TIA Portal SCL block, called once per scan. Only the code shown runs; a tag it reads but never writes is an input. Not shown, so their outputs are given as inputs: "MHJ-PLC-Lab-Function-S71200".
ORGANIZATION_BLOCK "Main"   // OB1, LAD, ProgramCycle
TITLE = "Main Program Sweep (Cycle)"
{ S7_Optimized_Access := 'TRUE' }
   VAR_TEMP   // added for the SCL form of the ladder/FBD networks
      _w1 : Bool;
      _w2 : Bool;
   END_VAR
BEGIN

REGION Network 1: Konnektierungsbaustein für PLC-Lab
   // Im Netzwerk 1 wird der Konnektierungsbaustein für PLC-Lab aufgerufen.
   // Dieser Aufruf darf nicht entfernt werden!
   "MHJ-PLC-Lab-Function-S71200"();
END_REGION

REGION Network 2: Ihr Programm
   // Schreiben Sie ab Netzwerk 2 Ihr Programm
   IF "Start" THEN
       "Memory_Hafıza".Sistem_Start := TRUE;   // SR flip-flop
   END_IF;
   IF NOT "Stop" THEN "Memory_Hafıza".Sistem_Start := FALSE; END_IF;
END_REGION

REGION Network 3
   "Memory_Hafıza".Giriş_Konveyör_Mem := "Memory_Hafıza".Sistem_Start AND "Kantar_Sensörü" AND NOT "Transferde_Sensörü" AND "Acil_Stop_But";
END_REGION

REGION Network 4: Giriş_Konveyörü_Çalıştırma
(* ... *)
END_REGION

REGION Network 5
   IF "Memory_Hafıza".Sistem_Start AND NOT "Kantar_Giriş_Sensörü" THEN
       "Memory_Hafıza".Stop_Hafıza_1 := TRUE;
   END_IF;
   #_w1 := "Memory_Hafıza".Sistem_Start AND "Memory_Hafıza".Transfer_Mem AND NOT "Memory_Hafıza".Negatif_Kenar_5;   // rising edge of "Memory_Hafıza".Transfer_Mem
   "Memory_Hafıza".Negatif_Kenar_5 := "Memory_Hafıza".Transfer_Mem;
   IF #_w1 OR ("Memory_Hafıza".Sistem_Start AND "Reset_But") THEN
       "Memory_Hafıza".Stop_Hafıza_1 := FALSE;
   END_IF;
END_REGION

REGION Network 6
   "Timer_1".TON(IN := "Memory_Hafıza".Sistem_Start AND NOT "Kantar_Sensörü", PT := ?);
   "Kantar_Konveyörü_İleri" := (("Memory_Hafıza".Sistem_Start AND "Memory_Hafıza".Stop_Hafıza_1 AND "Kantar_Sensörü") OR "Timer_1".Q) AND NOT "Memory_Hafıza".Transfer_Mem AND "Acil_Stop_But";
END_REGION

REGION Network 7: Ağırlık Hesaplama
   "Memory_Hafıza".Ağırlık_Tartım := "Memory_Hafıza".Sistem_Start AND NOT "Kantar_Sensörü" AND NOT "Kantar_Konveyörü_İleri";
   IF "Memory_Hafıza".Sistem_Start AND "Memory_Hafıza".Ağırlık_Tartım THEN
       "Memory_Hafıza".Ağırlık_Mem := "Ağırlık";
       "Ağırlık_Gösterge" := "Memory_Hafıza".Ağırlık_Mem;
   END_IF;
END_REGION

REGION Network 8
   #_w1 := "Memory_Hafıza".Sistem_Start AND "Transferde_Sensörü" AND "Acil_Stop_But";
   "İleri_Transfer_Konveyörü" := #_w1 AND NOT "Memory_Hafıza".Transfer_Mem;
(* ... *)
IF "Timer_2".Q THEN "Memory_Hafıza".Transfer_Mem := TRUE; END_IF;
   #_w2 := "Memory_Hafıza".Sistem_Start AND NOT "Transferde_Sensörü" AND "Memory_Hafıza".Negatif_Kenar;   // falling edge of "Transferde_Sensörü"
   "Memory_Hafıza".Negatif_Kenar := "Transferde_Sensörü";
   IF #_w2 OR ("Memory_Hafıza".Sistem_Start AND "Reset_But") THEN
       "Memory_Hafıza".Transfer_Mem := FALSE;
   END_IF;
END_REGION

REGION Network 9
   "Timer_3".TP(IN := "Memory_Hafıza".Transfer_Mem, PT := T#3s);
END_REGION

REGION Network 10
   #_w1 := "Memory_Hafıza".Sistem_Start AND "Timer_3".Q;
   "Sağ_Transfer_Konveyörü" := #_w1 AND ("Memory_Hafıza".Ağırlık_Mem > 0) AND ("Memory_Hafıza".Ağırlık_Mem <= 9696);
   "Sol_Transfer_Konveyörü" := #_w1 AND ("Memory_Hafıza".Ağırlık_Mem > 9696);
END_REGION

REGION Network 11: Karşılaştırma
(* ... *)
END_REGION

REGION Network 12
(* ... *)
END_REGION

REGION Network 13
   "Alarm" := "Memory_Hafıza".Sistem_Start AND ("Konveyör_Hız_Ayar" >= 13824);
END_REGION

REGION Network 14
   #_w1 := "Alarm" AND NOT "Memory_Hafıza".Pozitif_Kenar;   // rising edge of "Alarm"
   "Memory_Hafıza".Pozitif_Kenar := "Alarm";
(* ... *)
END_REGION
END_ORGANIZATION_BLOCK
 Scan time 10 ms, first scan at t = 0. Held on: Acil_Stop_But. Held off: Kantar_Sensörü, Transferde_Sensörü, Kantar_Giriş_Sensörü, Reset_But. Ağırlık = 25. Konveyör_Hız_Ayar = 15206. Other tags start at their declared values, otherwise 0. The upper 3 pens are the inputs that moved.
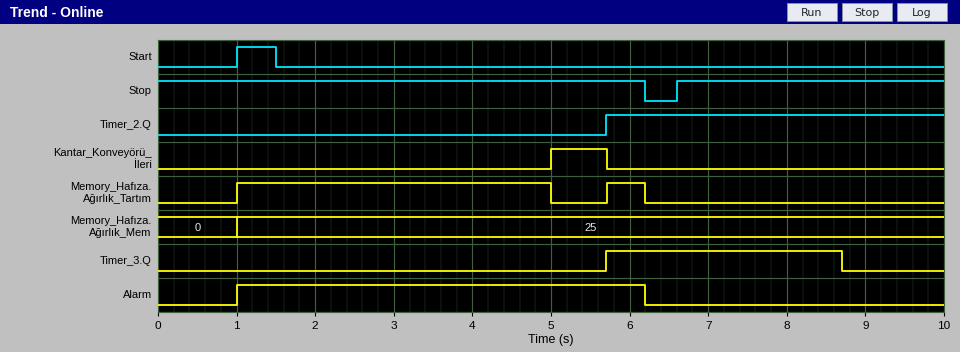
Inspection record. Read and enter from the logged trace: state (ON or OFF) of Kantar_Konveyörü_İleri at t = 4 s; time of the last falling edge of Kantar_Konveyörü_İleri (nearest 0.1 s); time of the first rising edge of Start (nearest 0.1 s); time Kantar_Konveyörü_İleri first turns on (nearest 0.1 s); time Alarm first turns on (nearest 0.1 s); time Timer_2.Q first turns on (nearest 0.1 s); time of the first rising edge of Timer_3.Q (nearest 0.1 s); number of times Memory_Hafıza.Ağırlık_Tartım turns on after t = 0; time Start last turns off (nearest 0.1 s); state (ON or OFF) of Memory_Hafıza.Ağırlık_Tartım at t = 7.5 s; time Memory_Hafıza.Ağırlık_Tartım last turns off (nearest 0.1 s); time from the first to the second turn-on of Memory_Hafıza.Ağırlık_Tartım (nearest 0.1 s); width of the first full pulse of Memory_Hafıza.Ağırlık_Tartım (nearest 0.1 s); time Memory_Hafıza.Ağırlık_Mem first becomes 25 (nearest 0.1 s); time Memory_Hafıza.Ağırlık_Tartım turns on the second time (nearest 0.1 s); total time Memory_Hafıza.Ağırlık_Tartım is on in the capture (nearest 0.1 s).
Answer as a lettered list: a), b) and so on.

a) OFF
b) 5.7 s
c) 1.0 s
d) 5.0 s
e) 1.0 s
f) 5.7 s
g) 5.7 s
h) 2
i) 1.5 s
j) OFF
k) 6.2 s
l) 4.7 s
m) 4.0 s
n) 1.0 s
o) 5.7 s
p) 4.5 s
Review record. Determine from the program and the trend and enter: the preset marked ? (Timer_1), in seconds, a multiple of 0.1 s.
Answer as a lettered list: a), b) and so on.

a) 4.0 s
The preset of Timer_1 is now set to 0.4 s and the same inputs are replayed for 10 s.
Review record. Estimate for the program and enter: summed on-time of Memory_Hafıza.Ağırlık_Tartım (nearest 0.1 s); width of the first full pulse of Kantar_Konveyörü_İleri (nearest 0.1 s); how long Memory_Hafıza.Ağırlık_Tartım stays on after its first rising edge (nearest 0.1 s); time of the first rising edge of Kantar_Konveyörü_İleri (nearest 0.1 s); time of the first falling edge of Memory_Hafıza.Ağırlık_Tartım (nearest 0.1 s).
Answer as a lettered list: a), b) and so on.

a) 0.9 s
b) 4.3 s
c) 0.4 s
d) 1.4 s
e) 1.4 s
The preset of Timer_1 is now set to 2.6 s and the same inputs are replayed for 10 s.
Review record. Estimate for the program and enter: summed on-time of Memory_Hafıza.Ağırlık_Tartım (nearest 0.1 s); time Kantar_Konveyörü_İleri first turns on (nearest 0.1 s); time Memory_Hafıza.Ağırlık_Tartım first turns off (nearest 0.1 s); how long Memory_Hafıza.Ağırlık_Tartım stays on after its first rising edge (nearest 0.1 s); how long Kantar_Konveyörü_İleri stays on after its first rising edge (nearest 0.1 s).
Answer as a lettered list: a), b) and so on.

a) 3.1 s
b) 3.6 s
c) 3.6 s
d) 2.6 s
e) 2.1 s
